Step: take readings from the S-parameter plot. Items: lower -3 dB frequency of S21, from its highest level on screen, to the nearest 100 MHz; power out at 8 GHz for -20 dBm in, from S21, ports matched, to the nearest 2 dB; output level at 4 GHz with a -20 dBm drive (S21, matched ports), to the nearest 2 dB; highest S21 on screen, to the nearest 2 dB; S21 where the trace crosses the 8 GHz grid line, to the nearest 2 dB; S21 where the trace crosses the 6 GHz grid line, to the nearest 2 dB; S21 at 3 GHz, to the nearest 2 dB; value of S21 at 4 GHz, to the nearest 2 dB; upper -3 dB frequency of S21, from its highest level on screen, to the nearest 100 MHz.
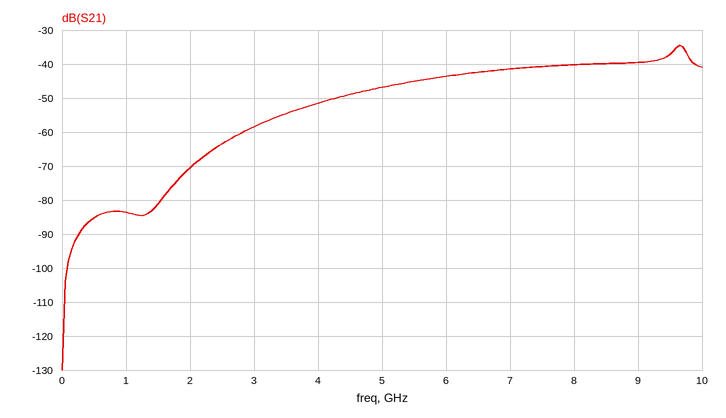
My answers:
9.5 GHz
-60 dBm
-72 dBm
-34 dB
-40 dB
-44 dB
-58 dB
-52 dB
9.8 GHz
